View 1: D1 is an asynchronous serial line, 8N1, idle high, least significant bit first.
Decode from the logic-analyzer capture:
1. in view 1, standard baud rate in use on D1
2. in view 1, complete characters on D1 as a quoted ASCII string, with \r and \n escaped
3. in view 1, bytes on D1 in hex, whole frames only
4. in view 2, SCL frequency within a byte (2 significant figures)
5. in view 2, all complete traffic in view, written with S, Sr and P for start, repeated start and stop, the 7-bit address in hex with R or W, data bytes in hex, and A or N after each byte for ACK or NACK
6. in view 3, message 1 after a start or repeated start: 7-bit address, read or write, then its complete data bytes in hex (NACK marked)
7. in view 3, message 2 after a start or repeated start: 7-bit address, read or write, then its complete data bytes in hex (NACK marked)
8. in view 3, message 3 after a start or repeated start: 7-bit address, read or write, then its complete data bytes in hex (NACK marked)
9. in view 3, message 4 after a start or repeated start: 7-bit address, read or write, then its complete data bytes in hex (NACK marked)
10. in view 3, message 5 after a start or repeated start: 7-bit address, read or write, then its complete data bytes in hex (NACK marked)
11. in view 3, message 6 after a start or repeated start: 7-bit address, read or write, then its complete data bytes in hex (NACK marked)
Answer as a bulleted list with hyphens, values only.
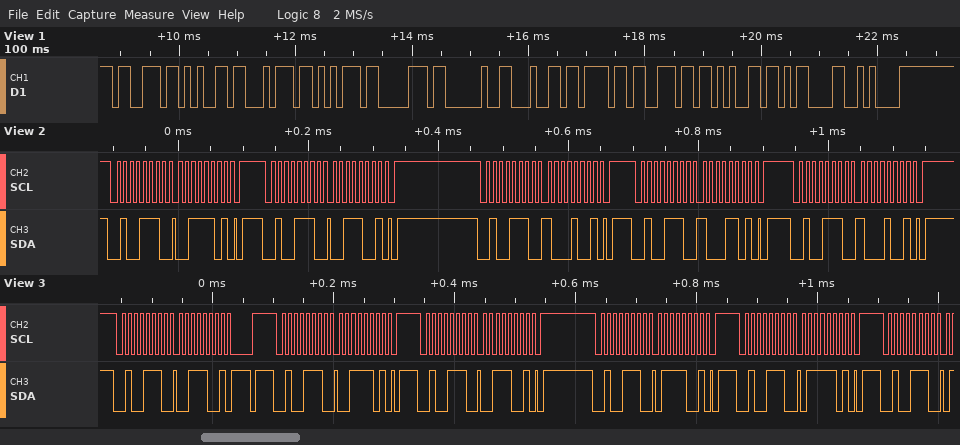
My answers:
- 9600 baud
- "setup done\r\n"
- 0x73 0x65 0x74 0x75 0x70 0x20 0x64 0x6F 0x6E 0x65 0x0D 0x0A
- 100 kHz
- S 27W A 3D A P S 27W A 39 A P S 27W A 89 A P S 27W A 8D A P S 27W A 89 A P
- 0x27 write: 39
- 0x27 write: 3D
- 0x27 write: 39
- 0x27 write: 79
- 0x27 write: 7D
- 0x27 write
